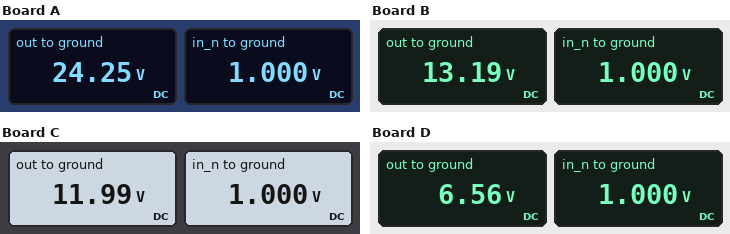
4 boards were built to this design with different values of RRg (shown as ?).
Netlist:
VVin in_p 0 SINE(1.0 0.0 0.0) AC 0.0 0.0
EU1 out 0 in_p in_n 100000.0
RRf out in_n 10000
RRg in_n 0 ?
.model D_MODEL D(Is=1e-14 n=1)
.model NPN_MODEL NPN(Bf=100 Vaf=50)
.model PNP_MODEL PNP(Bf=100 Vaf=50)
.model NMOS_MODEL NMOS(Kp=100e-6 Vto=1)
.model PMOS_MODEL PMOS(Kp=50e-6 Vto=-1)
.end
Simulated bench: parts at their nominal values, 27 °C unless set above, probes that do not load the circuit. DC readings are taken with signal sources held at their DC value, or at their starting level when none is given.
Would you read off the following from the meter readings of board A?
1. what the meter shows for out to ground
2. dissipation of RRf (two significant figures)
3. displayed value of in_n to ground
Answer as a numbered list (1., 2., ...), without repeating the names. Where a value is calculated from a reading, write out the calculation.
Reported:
1. 24.25 V
2. (24.25 V - 1 V)^2 / 10 kΩ = 54 mW
3. 1.000 V
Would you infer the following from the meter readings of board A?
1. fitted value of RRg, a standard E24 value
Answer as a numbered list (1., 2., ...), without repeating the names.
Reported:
1. 430 Ω
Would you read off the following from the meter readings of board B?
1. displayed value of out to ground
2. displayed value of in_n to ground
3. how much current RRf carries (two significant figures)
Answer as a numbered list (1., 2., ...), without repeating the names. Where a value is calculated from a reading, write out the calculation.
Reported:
1. 13.19 V
2. 1.000 V
3. (13.19 V - 1 V) / 10 kΩ = 1.2 mA
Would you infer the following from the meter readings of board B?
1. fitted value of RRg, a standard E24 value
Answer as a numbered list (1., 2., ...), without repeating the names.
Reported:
1. 820 Ω
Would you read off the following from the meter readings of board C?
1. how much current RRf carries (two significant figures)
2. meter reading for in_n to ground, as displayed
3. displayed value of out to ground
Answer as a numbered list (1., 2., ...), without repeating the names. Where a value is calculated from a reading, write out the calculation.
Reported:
1. (11.99 V - 1 V) / 10 kΩ = 1.1 mA
2. 1.000 V
3. 11.99 V
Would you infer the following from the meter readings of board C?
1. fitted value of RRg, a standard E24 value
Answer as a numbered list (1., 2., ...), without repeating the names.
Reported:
1. 910 Ω
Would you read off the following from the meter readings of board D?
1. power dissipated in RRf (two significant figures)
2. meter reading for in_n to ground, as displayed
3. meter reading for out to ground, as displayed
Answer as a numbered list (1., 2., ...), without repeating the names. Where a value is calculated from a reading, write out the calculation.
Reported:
1. (6.56 V - 1 V)^2 / 10 kΩ = 3.1 mW
2. 1.000 V
3. 6.56 V
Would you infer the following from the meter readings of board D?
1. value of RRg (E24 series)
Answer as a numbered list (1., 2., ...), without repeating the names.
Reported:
1. 1.8 kΩ
